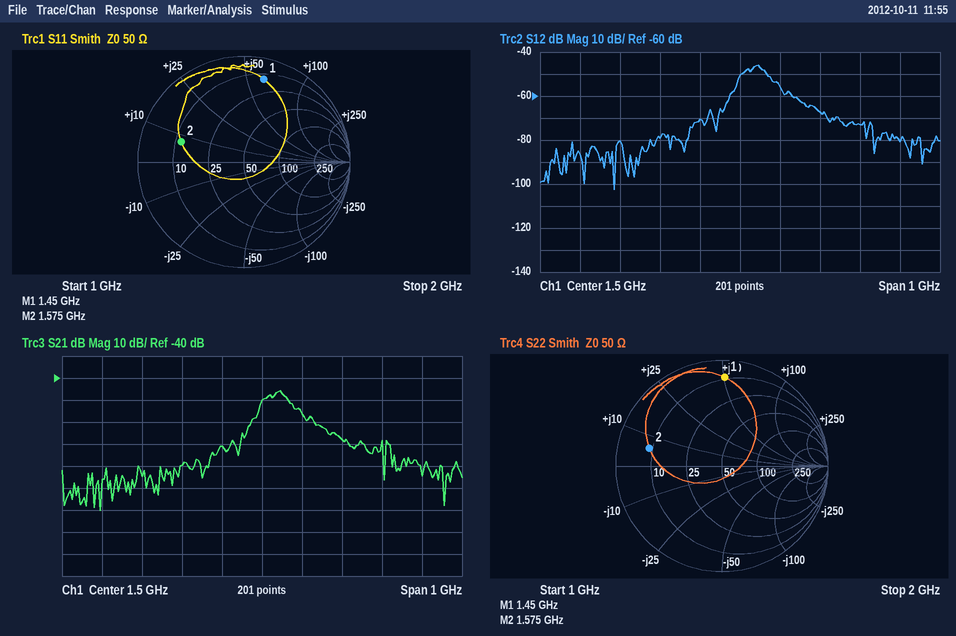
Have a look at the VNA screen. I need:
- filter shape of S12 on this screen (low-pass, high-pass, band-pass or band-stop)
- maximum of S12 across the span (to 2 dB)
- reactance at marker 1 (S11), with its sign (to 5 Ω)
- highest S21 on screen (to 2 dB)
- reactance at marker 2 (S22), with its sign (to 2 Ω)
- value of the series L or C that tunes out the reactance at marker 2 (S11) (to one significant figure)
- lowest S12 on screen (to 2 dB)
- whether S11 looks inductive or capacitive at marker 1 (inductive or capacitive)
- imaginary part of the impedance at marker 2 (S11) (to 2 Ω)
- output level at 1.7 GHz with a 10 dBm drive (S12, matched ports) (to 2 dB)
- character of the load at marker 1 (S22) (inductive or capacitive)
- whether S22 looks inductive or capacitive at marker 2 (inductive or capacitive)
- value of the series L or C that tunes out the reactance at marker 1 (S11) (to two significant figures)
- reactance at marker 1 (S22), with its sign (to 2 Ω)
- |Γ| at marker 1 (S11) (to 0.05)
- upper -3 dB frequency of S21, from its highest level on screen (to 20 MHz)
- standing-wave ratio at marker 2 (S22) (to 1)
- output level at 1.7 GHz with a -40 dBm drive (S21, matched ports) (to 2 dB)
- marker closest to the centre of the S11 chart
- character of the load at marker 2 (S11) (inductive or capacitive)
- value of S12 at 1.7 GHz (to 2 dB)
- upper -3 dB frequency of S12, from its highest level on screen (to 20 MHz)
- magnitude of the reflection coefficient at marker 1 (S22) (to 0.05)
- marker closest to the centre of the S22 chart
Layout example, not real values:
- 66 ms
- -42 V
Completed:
- band-pass
- -46 dB
- +60 Ω
- -46 dB
- +6 Ω
- 10 pF
- -102 dB
- inductive
- +8 Ω
- -58 dBm
- inductive
- inductive
- 1.8 pF
- +50 Ω
- 0.80
- 1.56 GHz
- 6
- -108 dBm
- marker 2
- inductive
- -68 dB
- 1.56 GHz
- 0.85
- marker 2
